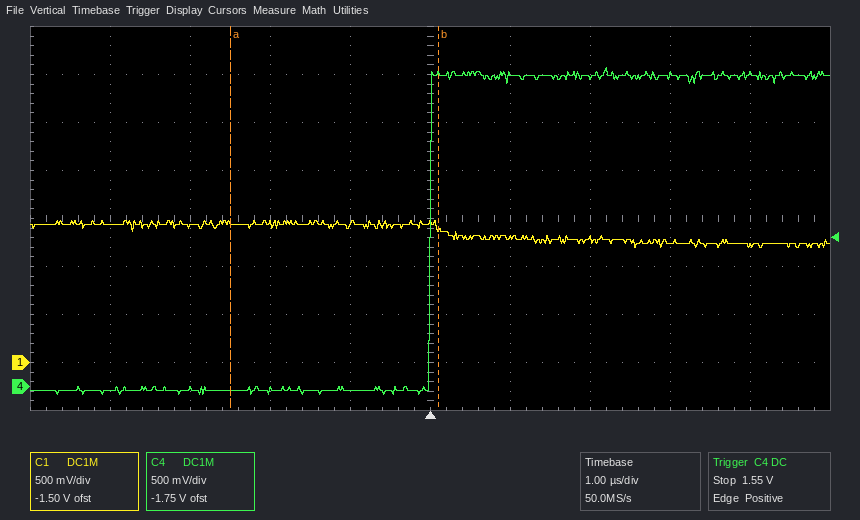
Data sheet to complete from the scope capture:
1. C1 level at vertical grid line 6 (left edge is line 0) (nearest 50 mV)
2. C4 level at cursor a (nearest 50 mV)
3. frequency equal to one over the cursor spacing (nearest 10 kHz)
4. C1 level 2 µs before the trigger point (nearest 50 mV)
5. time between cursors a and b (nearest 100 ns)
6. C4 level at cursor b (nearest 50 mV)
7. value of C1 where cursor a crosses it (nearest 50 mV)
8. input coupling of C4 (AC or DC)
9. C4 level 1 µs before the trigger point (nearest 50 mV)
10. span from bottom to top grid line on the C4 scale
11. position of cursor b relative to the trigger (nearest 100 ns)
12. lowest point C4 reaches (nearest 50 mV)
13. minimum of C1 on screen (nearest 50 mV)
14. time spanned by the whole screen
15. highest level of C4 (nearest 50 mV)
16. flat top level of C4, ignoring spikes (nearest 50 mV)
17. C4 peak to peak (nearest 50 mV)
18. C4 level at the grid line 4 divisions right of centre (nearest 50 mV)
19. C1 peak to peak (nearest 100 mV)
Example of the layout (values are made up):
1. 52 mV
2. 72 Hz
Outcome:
1. 1.30 V
2. -50 mV
3. 380 kHz
4. 1.45 V
5. 2.6 µs
6. 3.25 V
7. 1.45 V
8. DC
9. -50 mV
10. 4 V
11. +100 ns
12. -100 mV
13. 1.20 V
14. 10 µs
15. 3.30 V
16. 3.25 V
17. 3.40 V
18. 3.25 V
19. 300 mV
